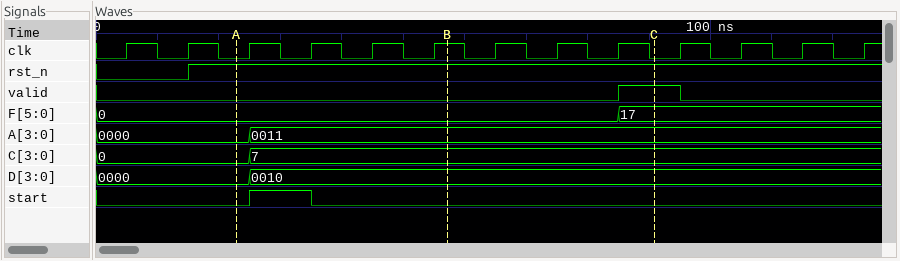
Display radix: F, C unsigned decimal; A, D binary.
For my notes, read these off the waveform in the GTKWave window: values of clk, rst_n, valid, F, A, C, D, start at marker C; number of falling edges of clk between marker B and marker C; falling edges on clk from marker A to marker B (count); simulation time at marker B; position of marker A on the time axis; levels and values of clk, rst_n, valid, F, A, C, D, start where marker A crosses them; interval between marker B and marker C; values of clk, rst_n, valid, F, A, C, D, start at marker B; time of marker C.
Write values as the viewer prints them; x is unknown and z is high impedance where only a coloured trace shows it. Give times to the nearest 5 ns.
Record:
clk=0, rst_n=1, valid=1, F=17, A=0011, C=7, D=0010, start=0
4
3
55 ns
25 ns
clk=0, rst_n=1, valid=0, F=0, A=0000, C=0, D=0000, start=0
35 ns
clk=1, rst_n=1, valid=0, F=0, A=0011, C=7, D=0010, start=0
90 ns
